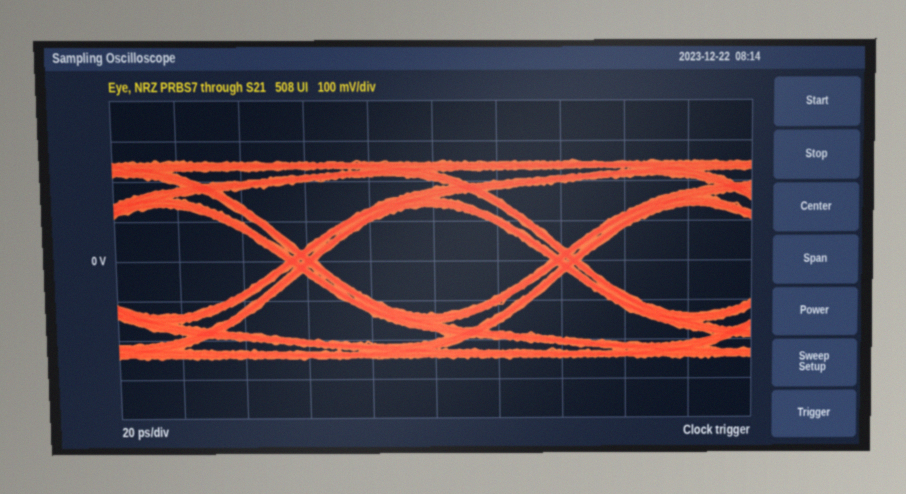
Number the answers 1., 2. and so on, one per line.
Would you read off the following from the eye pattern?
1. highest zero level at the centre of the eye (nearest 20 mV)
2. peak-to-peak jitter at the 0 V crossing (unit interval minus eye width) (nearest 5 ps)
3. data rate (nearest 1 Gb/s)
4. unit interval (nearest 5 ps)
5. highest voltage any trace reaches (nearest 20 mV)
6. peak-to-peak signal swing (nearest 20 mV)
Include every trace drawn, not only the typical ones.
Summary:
1. -140 mV
2. 10 ps
3. 12 Gb/s
4. 85 ps
5. 260 mV
6. 500 mV
